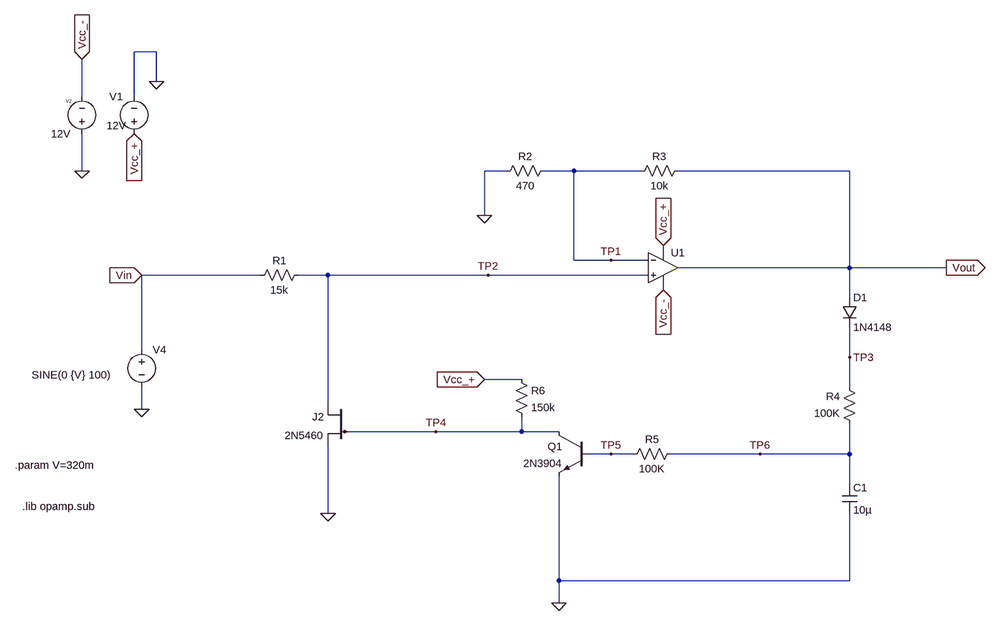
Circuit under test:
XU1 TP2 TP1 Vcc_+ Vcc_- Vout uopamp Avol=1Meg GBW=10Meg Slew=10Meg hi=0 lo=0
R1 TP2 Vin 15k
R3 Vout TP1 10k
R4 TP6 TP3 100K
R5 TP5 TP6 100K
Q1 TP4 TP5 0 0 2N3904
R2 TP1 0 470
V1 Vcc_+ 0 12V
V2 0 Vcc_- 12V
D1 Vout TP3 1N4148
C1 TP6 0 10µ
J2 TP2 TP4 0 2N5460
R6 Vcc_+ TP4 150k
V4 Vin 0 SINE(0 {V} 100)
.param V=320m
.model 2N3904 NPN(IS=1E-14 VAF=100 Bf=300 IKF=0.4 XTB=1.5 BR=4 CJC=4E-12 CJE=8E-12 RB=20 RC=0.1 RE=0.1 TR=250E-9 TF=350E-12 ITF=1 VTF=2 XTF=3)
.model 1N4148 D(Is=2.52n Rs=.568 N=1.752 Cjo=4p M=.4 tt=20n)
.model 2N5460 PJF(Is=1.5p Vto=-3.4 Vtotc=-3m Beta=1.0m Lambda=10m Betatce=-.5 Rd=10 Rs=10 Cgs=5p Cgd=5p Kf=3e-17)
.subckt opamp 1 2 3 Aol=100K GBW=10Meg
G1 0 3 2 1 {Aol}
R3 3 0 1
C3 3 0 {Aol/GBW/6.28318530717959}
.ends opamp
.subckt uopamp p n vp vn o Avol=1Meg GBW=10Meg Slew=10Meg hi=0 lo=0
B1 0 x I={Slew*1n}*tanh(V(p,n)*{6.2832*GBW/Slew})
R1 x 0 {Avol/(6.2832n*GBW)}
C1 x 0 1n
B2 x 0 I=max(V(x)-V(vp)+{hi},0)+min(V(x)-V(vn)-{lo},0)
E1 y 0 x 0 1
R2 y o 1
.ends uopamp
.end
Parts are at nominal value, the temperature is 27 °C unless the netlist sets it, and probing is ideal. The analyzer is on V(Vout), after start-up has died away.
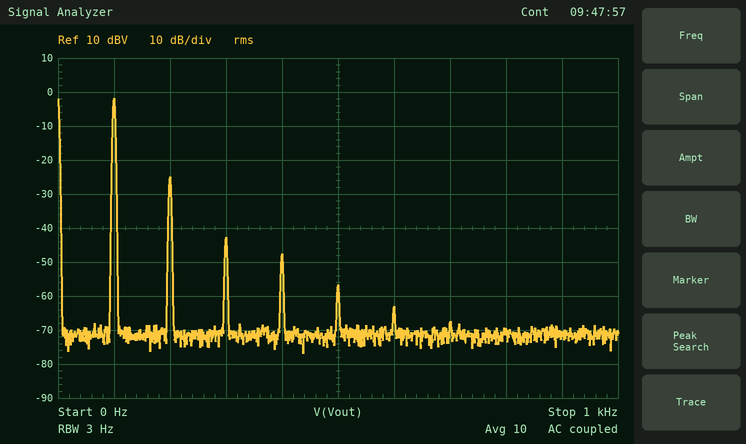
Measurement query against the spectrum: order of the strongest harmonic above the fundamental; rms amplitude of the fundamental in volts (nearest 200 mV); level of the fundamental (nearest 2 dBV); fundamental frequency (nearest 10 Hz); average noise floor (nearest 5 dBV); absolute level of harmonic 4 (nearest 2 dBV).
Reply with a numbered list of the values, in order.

1. 2
2. 800 mV
3. -2 dBV
4. 100 Hz
5. -70 dBV
6. -48 dBV
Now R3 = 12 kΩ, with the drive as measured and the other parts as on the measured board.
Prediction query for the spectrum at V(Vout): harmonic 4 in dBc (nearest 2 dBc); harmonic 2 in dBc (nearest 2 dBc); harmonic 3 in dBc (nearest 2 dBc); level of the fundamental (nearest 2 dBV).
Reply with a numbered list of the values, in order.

1. -48 dBc
2. -26 dBc
3. -42 dBc
4. -2 dBV
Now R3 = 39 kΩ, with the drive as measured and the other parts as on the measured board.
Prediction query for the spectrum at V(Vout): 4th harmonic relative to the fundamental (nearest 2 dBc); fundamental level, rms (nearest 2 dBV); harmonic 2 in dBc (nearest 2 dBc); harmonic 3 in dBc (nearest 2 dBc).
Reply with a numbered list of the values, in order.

1. -56 dBc
2. -2 dBV
3. -42 dBc
4. -50 dBc
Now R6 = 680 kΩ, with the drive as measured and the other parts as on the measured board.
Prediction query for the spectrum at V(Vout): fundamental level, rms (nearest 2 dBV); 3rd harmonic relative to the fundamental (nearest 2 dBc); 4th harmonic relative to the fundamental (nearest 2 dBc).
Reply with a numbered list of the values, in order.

1. -4 dBV
2. -48 dBc
3. -56 dBc
